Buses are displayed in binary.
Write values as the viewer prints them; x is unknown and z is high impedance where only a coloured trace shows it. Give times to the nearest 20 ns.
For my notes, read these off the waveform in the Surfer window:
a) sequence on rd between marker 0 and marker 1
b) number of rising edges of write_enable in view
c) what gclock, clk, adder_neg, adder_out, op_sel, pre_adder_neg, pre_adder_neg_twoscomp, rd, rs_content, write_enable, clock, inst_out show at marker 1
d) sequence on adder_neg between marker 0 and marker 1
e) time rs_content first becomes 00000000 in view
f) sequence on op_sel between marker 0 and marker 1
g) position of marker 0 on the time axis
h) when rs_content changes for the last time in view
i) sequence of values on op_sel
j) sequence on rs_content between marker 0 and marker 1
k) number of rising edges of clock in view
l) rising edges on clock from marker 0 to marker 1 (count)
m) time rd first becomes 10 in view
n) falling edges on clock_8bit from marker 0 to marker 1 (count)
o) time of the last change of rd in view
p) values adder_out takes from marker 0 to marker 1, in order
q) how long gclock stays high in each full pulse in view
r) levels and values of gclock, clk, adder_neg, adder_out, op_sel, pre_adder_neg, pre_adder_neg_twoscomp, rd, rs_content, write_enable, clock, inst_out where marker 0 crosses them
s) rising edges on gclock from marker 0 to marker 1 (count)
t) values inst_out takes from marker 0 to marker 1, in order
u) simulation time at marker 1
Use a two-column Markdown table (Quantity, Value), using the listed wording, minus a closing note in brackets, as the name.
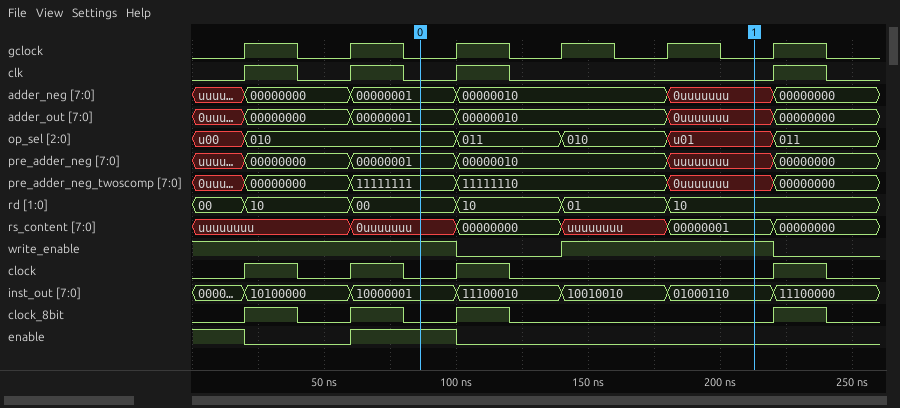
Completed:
| Quantity | Value |
|---|---|
| sequence on rd between marker 0 and marker 1 | 00, 10, 01, 10 |
| number of rising edges of write_enable in view | 1 |
| what gclock, clk, adder_neg, adder_out, op_sel, pre_adder_neg, pre_adder_neg_twoscomp, rd, rs_content, write_enable, clock, inst_out show at marker 1 | gclock=0, clk=0, adder_neg=0uuuuuuu, adder_out=0uuuuuuu, op_sel=u01, pre_adder_neg=uuuuuuuu, pre_adder_neg_twoscomp=0uuuuuuu, rd=10, rs_content=00000001, write_enable=1, clock=0, inst_out=01000110 |
| sequence on adder_neg between marker 0 and marker 1 | 00000001, 00000010, 0uuuuuuu |
| time rs_content first becomes 00000000 in view | 100 ns |
| sequence on op_sel between marker 0 and marker 1 | 010, 011, 010, u01 |
| position of marker 0 on the time axis | 80 ns |
| when rs_content changes for the last time in view | 220 ns |
| sequence of values on op_sel | u00, 010, 011, 010, u01, 011 |
| sequence on rs_content between marker 0 and marker 1 | 0uuuuuuu, 00000000, uuuuuuuu, 00000001 |
| number of rising edges of clock in view | 4 |
| rising edges on clock from marker 0 to marker 1 | 1 |
| time rd first becomes 10 in view | 20 ns |
| falling edges on clock_8bit from marker 0 to marker 1 | 1 |
| time of the last change of rd in view | 180 ns |
| values adder_out takes from marker 0 to marker 1, in order | 00000001, 00000010, 0uuuuuuu |
| how long gclock stays high in each full pulse in view | 20 ns, 20 ns, 20 ns, 20 ns, 20 ns, 20 ns |
| levels and values of gclock, clk, adder_neg, adder_out, op_sel, pre_adder_neg, pre_adder_neg_twoscomp, rd, rs_content, write_enable, clock, inst_out where marker 0 crosses them | gclock=0, clk=0, adder_neg=00000001, adder_out=00000001, op_sel=010, pre_adder_neg=00000001, pre_adder_neg_twoscomp=11111111, rd=00, rs_content=0uuuuuuu, write_enable=1, clock=0, inst_out=10000001 |
| rising edges on gclock from marker 0 to marker 1 | 3 |
| values inst_out takes from marker 0 to marker 1, in order | 10000001, 11100010, 10010010, 01000110 |
| simulation time at marker 1 | 220 ns |
